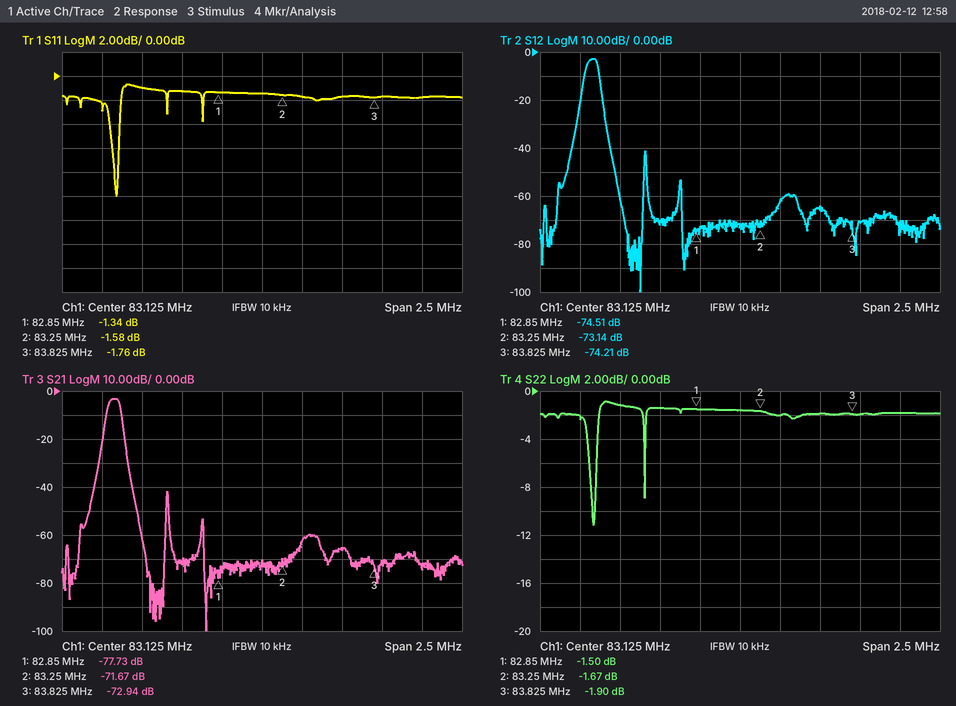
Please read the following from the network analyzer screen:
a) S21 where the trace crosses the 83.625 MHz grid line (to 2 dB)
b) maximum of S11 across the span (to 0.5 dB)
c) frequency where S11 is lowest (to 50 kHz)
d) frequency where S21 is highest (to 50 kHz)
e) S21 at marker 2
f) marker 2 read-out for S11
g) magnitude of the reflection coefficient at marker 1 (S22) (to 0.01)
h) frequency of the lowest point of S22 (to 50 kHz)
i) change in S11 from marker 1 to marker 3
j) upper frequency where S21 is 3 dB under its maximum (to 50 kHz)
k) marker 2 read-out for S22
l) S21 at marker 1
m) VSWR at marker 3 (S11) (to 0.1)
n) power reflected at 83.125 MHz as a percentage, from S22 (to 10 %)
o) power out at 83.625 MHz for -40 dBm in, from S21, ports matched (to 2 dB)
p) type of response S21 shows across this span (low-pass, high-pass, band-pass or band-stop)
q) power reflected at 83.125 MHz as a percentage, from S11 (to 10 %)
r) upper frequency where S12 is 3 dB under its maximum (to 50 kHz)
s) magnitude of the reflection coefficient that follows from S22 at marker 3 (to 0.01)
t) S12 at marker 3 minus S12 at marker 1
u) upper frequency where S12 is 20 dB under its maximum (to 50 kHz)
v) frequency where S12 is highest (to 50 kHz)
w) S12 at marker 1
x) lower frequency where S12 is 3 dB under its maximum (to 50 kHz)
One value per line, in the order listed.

-66 dB
-0.5 dB
82.20 MHz
82.20 MHz
-71.67 dB
-1.58 dB
0.84
82.20 MHz
-0.42 dB
82.25 MHz
-1.67 dB
-77.73 dB
9.9
70 %
-106 dBm
band-pass
70 %
82.25 MHz
0.80
0.30 dB
82.25 MHz
82.20 MHz
-74.51 dB
82.15 MHz
